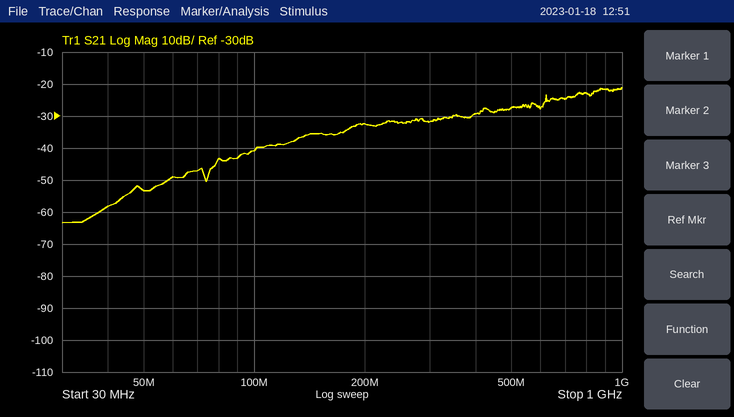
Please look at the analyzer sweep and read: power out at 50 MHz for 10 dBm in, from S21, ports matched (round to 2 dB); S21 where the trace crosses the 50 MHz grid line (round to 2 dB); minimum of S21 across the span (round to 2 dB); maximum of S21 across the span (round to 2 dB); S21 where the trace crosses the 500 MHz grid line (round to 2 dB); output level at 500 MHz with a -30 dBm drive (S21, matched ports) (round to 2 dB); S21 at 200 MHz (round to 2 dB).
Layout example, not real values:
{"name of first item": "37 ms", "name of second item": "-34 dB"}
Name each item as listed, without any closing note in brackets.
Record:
{"power out at 50 MHz for 10 dBm in, from S21, ports matched": "-44 dBm", "S21 where the trace crosses the 50 MHz grid line": "-54 dB", "minimum of S21 across the span": "-64 dB", "maximum of S21 across the span": "-22 dB", "S21 where the trace crosses the 500 MHz grid line": "-28 dB", "output level at 500 MHz with a -30 dBm drive (S21, matched ports)": "-58 dBm", "S21 at 200 MHz": "-32 dB"}
